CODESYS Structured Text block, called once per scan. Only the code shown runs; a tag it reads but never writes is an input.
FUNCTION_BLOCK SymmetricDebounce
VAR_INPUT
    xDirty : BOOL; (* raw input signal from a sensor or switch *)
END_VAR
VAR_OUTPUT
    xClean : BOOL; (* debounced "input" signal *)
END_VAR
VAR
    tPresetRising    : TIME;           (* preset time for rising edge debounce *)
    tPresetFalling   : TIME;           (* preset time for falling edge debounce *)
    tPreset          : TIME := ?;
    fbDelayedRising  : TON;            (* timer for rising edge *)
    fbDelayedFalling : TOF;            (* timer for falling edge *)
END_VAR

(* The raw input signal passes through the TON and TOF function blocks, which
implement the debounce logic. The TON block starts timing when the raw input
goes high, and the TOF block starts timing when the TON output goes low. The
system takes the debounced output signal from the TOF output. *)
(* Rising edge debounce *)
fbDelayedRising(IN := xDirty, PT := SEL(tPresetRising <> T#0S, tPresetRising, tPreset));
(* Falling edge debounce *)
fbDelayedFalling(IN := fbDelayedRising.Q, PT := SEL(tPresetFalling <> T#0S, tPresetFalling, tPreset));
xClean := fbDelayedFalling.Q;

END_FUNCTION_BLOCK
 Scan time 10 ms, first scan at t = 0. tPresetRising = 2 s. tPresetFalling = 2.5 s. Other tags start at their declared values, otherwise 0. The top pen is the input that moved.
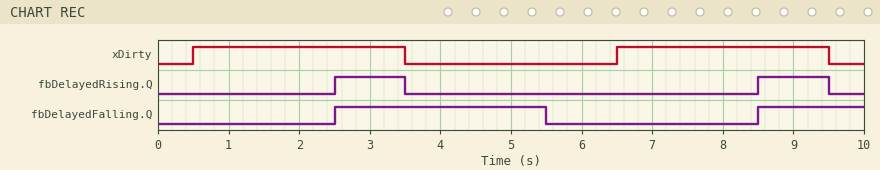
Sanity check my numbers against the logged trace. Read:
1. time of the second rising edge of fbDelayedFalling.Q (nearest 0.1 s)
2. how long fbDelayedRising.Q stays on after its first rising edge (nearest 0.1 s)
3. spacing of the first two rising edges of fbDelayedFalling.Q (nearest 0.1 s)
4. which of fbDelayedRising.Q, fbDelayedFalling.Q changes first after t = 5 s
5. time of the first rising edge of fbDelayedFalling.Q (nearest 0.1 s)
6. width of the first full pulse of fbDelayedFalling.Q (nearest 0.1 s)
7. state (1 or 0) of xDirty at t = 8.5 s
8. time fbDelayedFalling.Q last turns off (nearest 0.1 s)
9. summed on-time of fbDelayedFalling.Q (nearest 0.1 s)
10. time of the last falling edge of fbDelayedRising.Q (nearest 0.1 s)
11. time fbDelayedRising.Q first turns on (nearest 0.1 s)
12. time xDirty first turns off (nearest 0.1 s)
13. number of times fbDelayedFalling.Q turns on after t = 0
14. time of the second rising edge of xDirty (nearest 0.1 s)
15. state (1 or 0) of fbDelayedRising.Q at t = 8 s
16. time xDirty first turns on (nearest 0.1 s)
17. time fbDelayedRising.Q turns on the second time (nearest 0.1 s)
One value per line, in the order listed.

8.5 s
1.0 s
6.0 s
fbDelayedFalling.Q
2.5 s
3.0 s
1
5.5 s
4.5 s
9.5 s
2.5 s
3.5 s
2
6.5 s
0
0.5 s
8.5 s
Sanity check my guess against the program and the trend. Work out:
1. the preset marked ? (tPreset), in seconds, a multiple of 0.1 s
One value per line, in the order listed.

2.0 s
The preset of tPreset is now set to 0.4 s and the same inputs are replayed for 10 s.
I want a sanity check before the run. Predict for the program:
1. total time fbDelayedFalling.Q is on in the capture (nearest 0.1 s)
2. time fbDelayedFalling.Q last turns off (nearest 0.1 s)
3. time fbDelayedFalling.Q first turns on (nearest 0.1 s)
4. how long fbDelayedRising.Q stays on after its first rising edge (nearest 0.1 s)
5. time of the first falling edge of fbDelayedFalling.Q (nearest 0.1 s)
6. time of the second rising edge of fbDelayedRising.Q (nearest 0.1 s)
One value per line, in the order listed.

6.0 s
9.9 s
0.9 s
2.6 s
3.9 s
6.9 s
